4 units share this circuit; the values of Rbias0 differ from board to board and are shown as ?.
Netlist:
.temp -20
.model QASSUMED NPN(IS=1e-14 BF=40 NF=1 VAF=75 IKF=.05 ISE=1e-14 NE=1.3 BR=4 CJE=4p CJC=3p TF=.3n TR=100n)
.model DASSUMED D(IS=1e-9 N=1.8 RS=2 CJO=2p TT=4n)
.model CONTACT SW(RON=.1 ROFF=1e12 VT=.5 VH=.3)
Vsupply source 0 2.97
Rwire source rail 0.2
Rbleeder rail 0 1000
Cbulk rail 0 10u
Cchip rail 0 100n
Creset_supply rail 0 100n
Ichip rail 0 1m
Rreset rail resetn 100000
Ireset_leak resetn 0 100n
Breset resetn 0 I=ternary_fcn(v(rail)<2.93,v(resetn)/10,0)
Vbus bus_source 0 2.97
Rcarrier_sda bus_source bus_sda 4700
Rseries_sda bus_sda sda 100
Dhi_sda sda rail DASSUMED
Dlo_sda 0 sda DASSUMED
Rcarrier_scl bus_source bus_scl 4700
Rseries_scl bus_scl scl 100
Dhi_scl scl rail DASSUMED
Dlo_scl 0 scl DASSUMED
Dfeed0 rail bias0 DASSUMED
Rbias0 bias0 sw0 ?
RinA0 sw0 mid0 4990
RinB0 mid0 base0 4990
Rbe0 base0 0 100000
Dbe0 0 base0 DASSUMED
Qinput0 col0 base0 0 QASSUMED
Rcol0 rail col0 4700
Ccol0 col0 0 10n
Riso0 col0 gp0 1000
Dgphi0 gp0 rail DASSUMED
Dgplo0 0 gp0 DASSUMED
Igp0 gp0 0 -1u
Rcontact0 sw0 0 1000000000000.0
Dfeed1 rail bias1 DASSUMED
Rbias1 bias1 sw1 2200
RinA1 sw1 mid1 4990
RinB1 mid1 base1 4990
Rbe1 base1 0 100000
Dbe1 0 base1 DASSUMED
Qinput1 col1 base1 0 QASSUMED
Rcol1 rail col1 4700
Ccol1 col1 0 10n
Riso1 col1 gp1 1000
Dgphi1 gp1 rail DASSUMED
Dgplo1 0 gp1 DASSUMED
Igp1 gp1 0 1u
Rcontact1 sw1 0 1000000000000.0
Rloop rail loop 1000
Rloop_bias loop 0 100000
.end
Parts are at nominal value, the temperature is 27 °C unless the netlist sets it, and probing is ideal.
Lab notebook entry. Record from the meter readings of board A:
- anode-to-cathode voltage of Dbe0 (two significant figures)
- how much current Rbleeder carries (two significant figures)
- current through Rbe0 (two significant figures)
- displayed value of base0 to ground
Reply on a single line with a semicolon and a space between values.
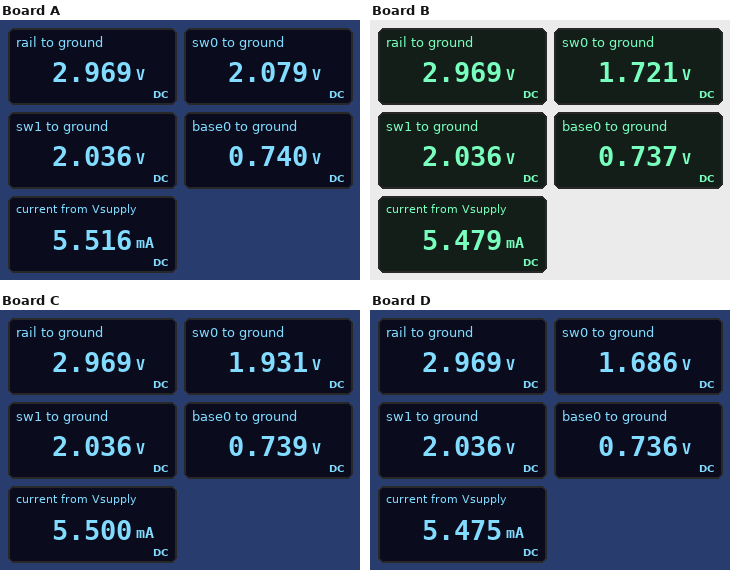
-740 mV; 3.0 mA; 7.4 µA; 0.740 V
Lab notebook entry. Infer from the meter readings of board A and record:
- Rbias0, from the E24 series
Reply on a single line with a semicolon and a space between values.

1.8 kΩ
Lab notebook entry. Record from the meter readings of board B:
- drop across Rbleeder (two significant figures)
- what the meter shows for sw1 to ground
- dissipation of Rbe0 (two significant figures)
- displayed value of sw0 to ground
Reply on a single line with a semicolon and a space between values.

3.0 V; 2.036 V; 5.4 µW; 1.721 V
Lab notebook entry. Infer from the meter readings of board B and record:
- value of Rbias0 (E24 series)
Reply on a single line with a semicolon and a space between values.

6.2 kΩ
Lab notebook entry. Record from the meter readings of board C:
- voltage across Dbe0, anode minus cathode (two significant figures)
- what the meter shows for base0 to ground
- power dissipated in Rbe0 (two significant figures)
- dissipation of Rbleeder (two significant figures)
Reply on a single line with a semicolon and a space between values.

-740 mV; 0.739 V; 5.5 µW; 8.8 mW
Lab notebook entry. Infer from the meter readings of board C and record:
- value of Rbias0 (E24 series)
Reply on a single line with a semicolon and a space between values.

3.3 kΩ
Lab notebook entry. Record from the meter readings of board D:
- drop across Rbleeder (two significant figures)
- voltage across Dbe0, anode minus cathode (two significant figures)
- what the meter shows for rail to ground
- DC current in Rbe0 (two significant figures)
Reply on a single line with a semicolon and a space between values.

3.0 V; -740 mV; 2.969 V; 7.4 µA
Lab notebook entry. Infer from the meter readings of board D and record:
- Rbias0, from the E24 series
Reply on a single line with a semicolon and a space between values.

6.8 kΩ
